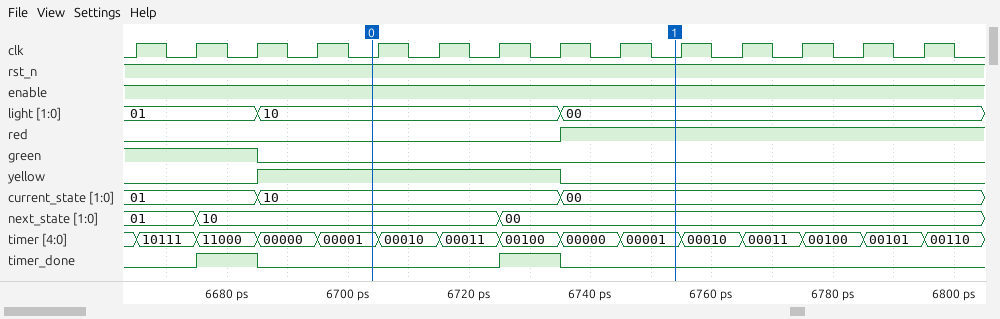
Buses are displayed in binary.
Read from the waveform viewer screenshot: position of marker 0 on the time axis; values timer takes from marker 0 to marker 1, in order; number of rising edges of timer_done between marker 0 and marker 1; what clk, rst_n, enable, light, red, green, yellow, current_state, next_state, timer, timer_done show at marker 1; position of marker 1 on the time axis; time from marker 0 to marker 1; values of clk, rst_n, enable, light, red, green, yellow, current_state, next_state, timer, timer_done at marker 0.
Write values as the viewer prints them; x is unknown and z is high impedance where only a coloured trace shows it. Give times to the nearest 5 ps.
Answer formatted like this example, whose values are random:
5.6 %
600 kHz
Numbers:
6705 ps
00001, 00010, 00011, 00100, 00000, 00001
1
clk=0, rst_n=1, enable=1, light=00, red=1, green=0, yellow=0, current_state=00, next_state=00, timer=00001, timer_done=0
6755 ps
50 ps
clk=0, rst_n=1, enable=1, light=10, red=0, green=0, yellow=1, current_state=10, next_state=10, timer=00001, timer_done=0
